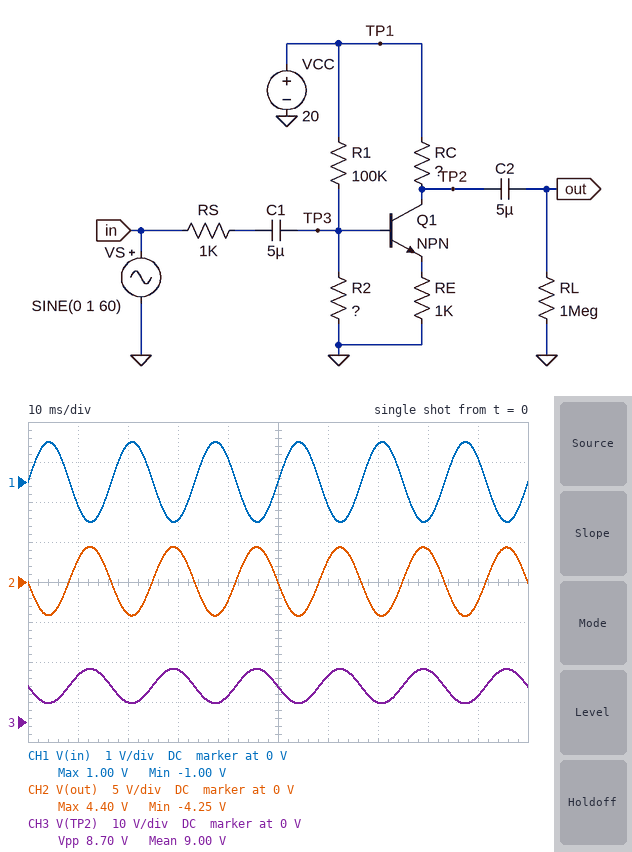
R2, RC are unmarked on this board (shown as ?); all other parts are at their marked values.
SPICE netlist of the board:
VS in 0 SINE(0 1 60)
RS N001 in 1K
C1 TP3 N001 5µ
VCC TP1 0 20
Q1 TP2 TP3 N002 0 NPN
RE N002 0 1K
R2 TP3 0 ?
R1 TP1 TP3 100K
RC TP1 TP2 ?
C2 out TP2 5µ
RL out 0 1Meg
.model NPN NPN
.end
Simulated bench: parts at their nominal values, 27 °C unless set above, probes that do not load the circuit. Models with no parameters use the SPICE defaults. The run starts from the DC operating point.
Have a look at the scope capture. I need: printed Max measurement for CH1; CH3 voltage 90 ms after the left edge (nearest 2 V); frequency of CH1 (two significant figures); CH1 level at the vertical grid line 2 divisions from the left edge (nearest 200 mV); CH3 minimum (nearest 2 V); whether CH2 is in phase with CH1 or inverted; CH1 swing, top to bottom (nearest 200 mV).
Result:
1.00 V
6 V
60 Hz
1.0 V
4 V
inverted
2.0 V
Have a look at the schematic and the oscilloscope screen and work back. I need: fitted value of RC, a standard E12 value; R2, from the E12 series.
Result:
4.7 kΩ
22 kΩ
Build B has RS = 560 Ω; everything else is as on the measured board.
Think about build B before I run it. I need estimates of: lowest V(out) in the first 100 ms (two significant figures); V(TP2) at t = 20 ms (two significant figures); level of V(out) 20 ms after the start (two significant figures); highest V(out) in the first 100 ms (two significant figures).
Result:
-4.4 V
4.8 V
-4.1 V
4.5 V
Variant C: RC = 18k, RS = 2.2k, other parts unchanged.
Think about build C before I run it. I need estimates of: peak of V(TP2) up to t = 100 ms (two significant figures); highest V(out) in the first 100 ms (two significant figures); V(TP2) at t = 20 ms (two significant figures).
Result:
15 V
14 V
1.4 V
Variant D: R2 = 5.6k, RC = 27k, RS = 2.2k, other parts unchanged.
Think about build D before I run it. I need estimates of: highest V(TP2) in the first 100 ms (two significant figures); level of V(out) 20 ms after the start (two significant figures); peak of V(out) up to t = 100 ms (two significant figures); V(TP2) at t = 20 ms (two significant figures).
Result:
20 V
-11 V
7.9 V
860 mV
